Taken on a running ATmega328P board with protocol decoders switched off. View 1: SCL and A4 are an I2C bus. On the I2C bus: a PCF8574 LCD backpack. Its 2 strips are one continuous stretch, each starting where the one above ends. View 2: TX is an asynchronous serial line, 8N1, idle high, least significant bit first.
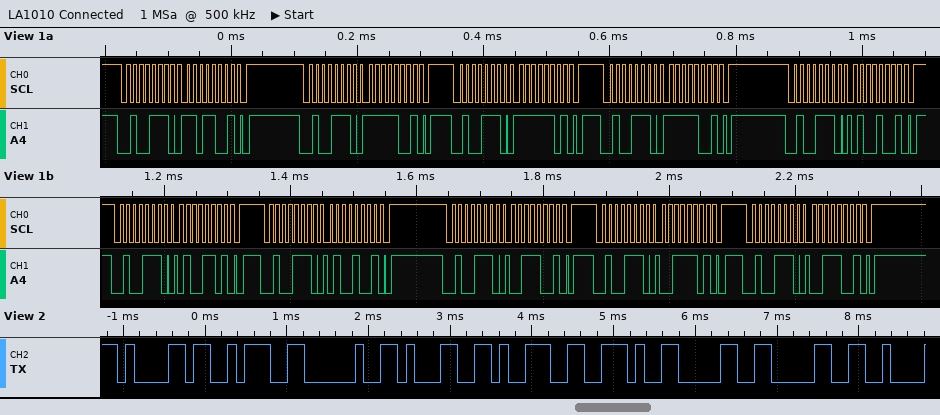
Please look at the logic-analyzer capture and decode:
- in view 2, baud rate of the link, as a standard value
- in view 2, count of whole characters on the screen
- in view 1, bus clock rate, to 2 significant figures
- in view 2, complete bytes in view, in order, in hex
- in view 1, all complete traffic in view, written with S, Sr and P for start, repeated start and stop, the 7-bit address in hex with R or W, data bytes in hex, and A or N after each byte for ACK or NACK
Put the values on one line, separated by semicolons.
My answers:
9600 baud; 8; 100 kHz; 61 3A 20 31 39 2E 30 30; S 27W A D9 A P S 27W A F9 A P S 27W A FD A P S 27W A F9 A P S 27W A 49 A P S 27W A 4D A P S 27W A 49 A P S 27W A 39 A P S 27W A 3D A P S 27W A 39 A P
